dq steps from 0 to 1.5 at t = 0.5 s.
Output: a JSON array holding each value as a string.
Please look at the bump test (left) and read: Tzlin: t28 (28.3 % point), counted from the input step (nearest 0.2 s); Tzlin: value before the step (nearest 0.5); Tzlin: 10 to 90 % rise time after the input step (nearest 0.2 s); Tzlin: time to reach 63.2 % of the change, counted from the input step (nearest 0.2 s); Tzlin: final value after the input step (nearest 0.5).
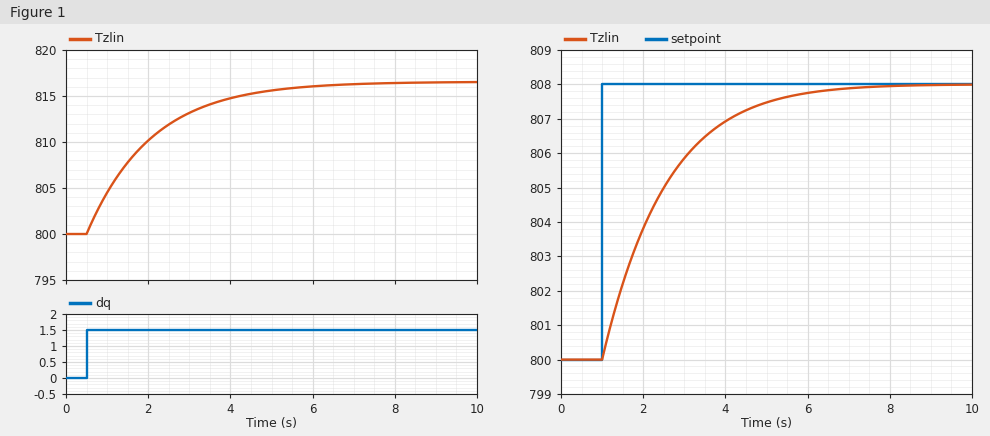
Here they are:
["0.6 s", "800.0", "3.4 s", "1.6 s", "816.5"]
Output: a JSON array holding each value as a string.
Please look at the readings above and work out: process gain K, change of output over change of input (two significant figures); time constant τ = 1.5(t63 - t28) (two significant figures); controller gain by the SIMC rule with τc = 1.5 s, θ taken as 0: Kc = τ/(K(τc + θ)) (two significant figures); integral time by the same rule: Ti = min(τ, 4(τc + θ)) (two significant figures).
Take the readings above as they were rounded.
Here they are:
["11", "1.5 s", "0.091", "1.5 s"]
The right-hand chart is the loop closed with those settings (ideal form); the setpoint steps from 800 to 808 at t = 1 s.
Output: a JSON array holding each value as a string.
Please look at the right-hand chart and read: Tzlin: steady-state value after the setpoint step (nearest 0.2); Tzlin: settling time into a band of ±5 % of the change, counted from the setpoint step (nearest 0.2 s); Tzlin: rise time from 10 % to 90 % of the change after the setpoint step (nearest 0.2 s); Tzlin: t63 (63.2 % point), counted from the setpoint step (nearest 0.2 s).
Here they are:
["808.0", "4.4 s", "3.2 s", "1.6 s"]
